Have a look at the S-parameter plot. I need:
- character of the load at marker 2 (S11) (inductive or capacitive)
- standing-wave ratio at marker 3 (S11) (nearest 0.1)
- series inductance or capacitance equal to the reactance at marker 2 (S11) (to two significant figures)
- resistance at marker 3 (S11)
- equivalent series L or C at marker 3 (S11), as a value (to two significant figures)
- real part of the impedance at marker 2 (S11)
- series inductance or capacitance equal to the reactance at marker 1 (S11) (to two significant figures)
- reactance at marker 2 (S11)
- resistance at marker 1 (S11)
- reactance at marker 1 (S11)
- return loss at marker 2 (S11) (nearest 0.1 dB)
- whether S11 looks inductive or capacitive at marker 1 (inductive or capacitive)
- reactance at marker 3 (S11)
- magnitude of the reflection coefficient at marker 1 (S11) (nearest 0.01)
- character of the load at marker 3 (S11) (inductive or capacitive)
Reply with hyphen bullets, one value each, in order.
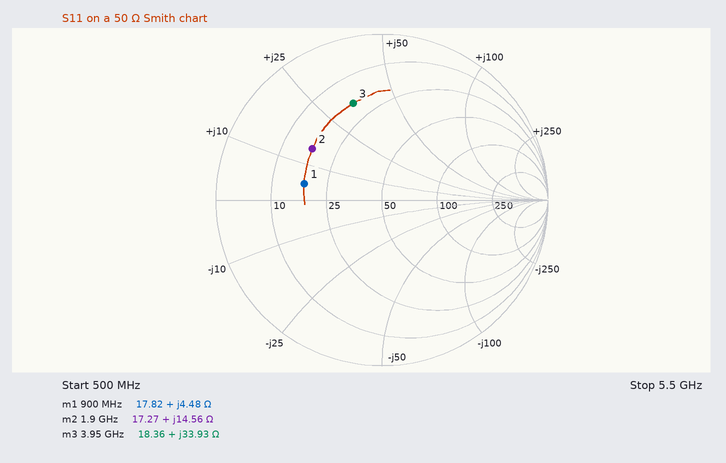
- inductive
- 4.1
- 1.2 nH
- 18.36 Ω
- 1.4 nH
- 17.27 Ω
- 790 pH
- +14.56 Ω
- 17.82 Ω
- +4.48 Ω
- 5.7 dB
- inductive
- +33.93 Ω
- 0.48
- inductive
